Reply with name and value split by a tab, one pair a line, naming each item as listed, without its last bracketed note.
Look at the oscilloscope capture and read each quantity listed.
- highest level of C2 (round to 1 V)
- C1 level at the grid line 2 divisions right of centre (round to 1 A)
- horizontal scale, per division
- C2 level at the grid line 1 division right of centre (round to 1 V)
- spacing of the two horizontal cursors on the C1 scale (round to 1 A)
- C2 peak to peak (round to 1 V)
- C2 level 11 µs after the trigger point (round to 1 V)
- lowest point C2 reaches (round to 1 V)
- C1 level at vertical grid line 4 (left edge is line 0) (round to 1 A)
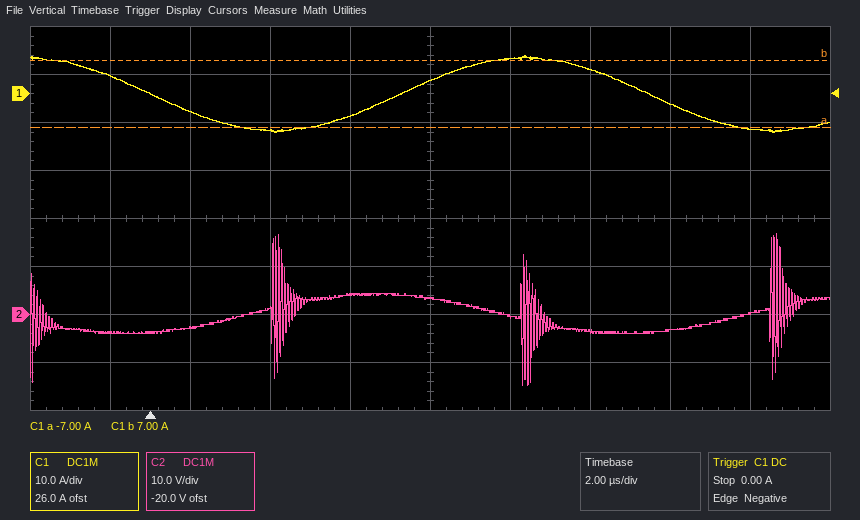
highest level of C2	17 V
C1 level at the grid line 2 divisions right of centre	5 A
horizontal scale, per division	2 µs
C2 level at the grid line 1 division right of centre	0 V
spacing of the two horizontal cursors on the C1 scale	14 A
C2 peak to peak	32 V
C2 level 11 µs after the trigger point	-4 V
lowest point C2 reaches	-15 V
C1 level at vertical grid line 4 (left edge is line 0)	-5 A
